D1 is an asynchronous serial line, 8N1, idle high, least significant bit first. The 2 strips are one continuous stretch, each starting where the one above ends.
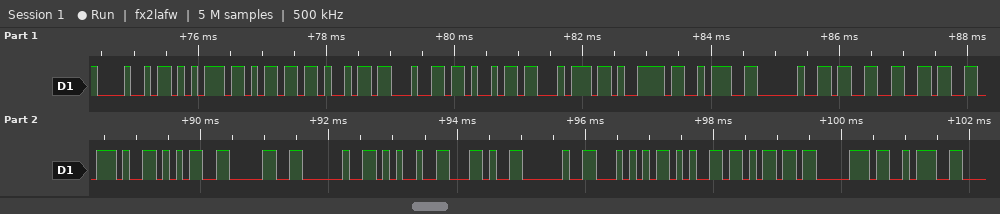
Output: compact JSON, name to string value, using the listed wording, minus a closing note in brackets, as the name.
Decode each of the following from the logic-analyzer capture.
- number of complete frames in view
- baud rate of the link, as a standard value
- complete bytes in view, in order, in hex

{"number of complete frames in view": "24", "baud rate of the link, as a standard value": "9600 baud", "complete bytes in view, in order, in hex": "48 75 6D 69 64 69 74 79 3A 20 33 36 2E 35 30 20 25 2C 20 54 65 6D 70 3A"}
